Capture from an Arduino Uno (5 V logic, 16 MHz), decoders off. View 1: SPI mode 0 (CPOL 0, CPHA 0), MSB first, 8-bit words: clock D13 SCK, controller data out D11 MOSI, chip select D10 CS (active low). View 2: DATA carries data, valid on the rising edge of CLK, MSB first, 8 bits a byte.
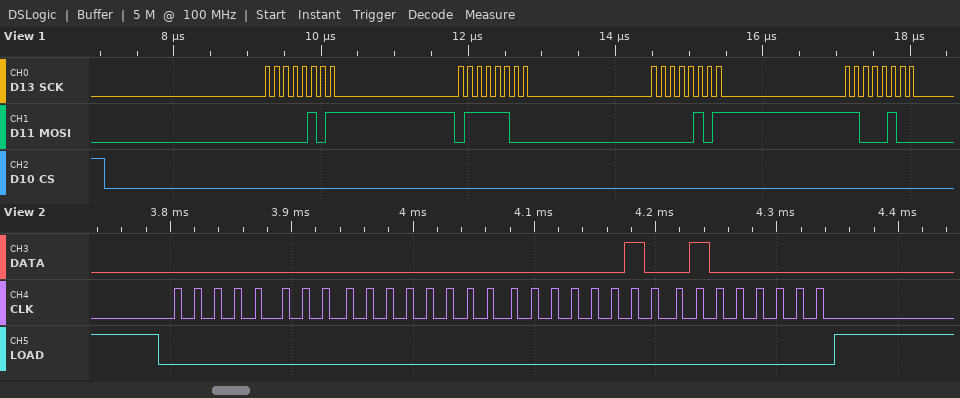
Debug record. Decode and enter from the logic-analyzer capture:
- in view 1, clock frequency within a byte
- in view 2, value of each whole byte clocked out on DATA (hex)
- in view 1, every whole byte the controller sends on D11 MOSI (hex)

8 MHz
0x00 0x00 0x02 0x40
05 7C 05 C4
